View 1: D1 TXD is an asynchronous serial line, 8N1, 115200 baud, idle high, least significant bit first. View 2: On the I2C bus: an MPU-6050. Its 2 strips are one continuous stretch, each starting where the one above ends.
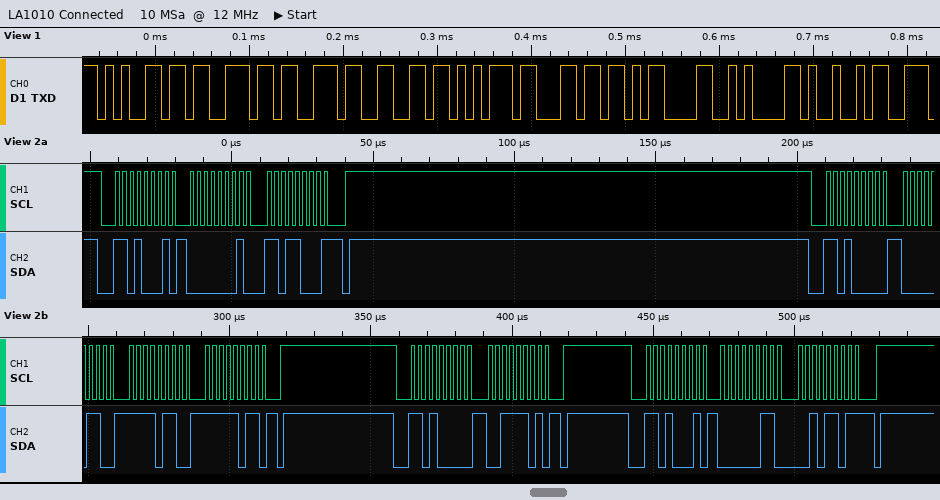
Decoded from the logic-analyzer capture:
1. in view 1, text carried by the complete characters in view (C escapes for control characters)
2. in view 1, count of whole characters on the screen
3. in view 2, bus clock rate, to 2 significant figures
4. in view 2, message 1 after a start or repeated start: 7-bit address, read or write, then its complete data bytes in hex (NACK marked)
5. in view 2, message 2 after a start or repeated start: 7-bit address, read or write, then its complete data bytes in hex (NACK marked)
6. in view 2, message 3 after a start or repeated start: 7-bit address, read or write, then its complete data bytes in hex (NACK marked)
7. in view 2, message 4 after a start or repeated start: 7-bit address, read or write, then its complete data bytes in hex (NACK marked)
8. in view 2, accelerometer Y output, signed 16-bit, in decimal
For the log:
"essful\r\nI"
9
400 kHz
0x68 read: 01 D8 NACK
0x68 write: 06 F6 FB
0x68 write: 3D
0x68 read: 03 2D NACK
813
